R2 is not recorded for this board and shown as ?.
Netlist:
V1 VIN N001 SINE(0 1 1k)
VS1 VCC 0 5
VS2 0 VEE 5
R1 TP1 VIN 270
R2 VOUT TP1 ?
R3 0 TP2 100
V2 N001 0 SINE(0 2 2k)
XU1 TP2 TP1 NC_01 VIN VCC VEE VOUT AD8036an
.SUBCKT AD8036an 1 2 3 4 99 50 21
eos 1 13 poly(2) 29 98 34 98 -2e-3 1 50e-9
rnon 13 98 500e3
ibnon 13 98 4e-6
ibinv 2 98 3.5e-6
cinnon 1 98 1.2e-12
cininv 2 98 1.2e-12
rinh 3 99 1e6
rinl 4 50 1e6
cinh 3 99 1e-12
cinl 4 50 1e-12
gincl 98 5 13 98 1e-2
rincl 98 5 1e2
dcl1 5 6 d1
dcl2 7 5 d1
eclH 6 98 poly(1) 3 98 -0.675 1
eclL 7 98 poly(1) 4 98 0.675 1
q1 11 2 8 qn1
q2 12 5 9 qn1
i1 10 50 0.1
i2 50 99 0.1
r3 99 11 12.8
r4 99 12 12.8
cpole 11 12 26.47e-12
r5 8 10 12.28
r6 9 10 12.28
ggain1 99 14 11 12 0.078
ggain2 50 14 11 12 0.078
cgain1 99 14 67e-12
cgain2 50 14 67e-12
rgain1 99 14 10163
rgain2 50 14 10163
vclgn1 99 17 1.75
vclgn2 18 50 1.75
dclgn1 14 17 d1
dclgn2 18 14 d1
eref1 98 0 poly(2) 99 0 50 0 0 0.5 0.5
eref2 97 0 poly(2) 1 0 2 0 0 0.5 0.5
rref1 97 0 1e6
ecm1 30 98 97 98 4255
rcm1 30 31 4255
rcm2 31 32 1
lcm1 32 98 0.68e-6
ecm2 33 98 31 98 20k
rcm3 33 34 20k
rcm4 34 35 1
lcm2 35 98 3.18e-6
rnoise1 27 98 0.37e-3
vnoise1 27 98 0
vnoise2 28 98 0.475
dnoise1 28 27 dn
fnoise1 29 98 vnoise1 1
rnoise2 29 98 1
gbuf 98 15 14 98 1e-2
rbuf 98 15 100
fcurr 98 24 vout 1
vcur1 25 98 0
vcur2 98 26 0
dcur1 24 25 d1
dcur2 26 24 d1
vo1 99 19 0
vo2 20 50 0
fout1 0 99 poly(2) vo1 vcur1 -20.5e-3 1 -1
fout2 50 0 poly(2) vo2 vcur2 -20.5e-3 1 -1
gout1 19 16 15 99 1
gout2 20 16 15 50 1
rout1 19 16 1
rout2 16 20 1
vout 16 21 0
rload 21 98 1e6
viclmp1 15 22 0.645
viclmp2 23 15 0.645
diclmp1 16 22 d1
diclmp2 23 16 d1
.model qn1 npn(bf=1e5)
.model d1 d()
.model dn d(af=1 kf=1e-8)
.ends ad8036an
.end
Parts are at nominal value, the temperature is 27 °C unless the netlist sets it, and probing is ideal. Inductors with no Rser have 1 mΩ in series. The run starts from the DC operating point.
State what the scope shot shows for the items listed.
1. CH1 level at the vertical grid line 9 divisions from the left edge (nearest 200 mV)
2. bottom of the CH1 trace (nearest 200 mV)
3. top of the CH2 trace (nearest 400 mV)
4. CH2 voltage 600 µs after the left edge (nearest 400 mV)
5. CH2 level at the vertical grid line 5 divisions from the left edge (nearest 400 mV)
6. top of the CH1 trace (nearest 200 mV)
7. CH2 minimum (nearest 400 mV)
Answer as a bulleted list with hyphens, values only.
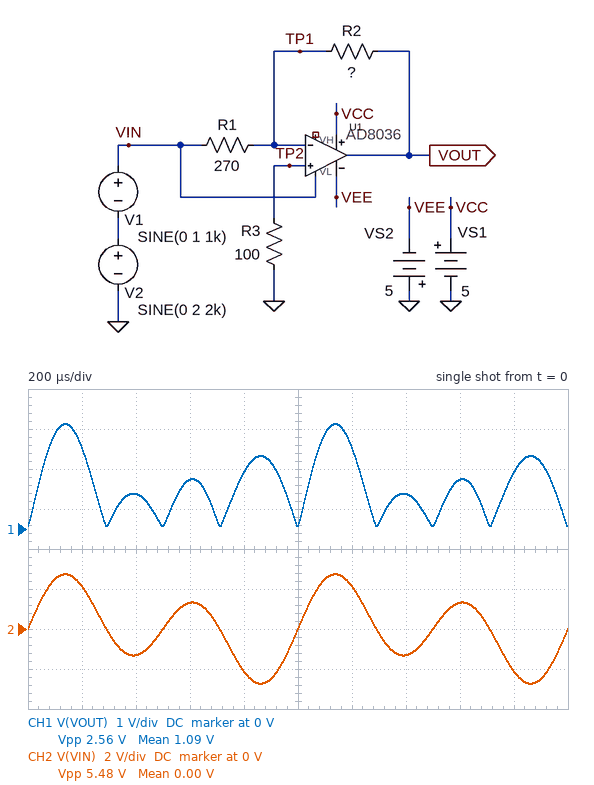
- 1.4 V
- 0 V
- 2.8 V
- 1.2 V
- 0 V
- 2.6 V
- -2.8 V
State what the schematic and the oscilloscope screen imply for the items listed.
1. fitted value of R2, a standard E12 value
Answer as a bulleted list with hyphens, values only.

- 180 Ω
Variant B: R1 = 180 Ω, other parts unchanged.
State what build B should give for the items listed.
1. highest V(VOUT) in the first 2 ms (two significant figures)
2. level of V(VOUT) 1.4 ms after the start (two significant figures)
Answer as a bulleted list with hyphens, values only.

- 2.7 V
- 1.3 V
